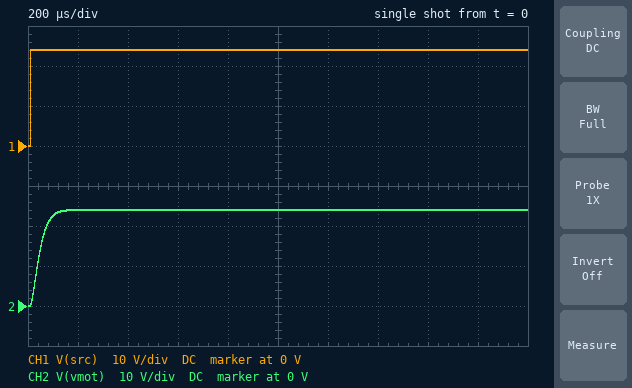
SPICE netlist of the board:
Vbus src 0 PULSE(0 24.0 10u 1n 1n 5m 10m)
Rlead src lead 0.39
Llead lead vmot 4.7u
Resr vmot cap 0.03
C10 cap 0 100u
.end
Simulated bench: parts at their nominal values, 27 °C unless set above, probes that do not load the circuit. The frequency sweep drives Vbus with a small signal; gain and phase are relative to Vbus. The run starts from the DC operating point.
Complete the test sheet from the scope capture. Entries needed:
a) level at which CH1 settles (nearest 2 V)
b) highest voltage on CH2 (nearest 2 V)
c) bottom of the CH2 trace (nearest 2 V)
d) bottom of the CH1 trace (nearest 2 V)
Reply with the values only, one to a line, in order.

24 V
24 V
0 V
0 V
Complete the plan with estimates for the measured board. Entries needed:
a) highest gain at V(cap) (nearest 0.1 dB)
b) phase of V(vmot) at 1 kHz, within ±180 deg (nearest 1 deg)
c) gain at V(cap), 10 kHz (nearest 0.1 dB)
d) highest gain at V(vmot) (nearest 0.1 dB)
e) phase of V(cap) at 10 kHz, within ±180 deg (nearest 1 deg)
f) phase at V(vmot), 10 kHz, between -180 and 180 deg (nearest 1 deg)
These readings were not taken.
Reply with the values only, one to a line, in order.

0 dB
-14 deg
-8.9 dB
0 dB
-108 deg
-97 deg
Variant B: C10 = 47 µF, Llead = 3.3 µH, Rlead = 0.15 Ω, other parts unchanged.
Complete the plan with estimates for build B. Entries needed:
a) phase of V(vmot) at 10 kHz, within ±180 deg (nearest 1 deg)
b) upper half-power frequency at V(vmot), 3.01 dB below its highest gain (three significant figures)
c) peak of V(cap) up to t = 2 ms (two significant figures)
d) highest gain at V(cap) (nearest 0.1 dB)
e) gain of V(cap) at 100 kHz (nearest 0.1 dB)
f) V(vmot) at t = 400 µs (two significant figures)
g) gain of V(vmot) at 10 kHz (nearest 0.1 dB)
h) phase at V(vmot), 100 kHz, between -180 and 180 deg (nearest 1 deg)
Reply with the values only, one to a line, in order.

-49 deg
15.2 kHz
32 V
3.9 dB
-35.6 dB
24 V
3.7 dB
-133 deg
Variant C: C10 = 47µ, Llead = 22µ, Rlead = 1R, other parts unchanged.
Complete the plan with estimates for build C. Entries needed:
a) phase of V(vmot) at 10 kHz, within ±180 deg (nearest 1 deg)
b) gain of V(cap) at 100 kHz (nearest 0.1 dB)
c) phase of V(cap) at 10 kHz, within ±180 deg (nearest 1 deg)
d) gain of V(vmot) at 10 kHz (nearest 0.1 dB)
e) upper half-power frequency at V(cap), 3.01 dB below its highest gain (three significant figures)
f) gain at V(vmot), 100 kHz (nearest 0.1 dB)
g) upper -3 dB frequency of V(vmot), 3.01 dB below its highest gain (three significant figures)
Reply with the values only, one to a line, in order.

-130 deg
-52.2 dB
-135 deg
-12.7 dB
4.63 kHz
-49.7 dB
4.64 kHz
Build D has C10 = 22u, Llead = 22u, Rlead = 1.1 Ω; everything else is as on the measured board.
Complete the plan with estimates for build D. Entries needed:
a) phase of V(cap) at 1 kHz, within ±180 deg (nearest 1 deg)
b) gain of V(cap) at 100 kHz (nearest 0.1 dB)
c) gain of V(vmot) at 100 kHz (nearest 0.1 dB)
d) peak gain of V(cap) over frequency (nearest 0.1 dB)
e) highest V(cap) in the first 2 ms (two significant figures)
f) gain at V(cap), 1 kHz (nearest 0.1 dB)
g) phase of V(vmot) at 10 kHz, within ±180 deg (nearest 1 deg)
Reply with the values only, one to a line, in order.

-9 deg
-45.6 dB
-44.9 dB
0.6 dB
27 V
0.1 dB
-118 deg
